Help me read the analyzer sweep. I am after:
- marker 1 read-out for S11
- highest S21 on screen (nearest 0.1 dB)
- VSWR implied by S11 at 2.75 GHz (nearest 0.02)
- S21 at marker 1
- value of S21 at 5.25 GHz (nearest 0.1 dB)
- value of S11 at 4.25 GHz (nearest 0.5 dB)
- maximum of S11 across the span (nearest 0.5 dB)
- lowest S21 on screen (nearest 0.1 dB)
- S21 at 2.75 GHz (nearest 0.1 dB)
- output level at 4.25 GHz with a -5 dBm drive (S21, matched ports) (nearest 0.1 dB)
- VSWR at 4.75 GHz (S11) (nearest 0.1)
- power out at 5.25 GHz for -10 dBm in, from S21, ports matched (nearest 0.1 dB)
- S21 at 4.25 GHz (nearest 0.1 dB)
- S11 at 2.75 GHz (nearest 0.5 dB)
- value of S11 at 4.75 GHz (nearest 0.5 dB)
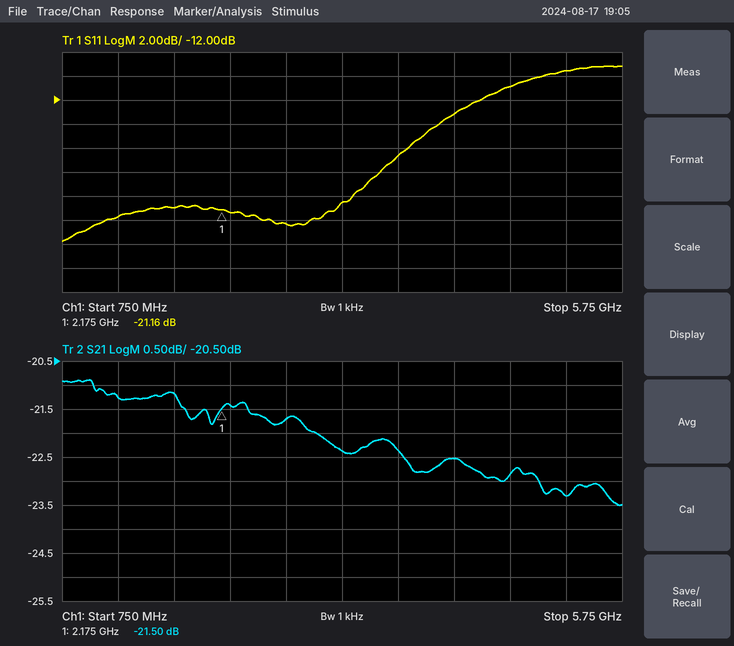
-21.16 dB
-20.9 dB
1.16
-21.50 dB
-23.3 dB
-13.0 dB
-9.0 dB
-23.5 dB
-21.7 dB
-27.5 dBm
1.8
-33.3 dBm
-22.5 dB
-22.5 dB
-11.0 dB
